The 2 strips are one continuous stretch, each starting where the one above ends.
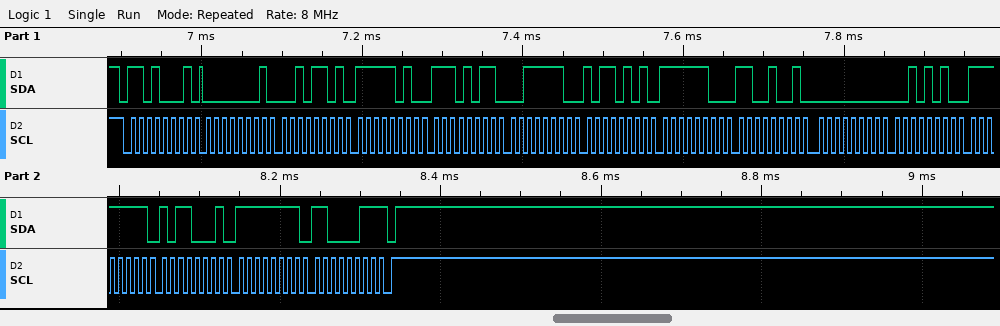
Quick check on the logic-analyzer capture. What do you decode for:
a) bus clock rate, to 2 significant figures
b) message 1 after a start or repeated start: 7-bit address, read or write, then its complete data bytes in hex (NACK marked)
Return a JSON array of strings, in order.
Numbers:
["100 kHz", "0x68 read: 01 2D FA EB 3E B5 FC C9 00 2A FF B1 FF C3 NACK"]
